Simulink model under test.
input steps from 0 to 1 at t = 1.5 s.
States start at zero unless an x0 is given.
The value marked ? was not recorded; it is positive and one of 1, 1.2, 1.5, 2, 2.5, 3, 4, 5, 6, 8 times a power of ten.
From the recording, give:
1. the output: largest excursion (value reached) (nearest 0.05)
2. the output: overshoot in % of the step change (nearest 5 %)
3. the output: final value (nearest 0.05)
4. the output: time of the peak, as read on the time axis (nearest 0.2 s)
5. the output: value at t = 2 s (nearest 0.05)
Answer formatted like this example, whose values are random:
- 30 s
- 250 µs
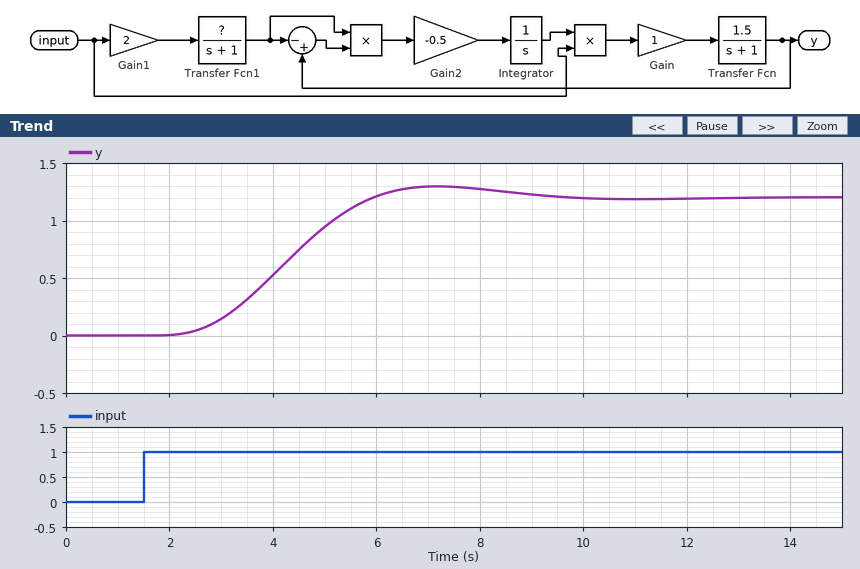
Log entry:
- 1.30
- 10 %
- 1.20
- 7.2 s
- 0.00
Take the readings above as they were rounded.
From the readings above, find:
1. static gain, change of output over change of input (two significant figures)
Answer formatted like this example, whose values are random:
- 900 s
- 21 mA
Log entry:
- 1.2
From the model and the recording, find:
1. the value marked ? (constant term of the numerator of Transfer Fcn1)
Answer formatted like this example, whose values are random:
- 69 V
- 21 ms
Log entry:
- 0.6
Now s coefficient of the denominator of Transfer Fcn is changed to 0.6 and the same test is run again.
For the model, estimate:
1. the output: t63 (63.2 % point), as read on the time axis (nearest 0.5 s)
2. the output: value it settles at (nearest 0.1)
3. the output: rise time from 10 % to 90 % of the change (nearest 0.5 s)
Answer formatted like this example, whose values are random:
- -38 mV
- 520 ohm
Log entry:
- 4.5 s
- 1.2
- 2.5 s
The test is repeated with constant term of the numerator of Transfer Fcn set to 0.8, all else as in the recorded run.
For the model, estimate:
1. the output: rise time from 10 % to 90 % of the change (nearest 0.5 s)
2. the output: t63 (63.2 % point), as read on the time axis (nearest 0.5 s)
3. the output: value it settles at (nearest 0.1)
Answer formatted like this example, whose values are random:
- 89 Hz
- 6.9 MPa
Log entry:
- 4.0 s
- 5.5 s
- 1.2
